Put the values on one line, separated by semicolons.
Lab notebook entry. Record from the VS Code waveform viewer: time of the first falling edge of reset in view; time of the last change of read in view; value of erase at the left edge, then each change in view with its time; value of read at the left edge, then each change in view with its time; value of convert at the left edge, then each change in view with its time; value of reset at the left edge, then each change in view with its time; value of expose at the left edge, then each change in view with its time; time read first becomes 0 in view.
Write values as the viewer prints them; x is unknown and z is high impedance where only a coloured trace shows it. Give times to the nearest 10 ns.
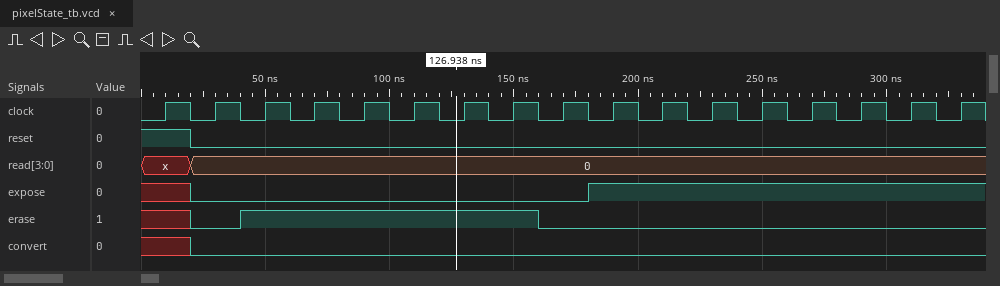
20 ns; 20 ns; x, 0 at 20 ns, 1 at 40 ns, 0 at 160 ns; x, 0 at 20 ns; x, 0 at 20 ns; 1, 0 at 20 ns; x, 0 at 20 ns, 1 at 180 ns; 20 ns
